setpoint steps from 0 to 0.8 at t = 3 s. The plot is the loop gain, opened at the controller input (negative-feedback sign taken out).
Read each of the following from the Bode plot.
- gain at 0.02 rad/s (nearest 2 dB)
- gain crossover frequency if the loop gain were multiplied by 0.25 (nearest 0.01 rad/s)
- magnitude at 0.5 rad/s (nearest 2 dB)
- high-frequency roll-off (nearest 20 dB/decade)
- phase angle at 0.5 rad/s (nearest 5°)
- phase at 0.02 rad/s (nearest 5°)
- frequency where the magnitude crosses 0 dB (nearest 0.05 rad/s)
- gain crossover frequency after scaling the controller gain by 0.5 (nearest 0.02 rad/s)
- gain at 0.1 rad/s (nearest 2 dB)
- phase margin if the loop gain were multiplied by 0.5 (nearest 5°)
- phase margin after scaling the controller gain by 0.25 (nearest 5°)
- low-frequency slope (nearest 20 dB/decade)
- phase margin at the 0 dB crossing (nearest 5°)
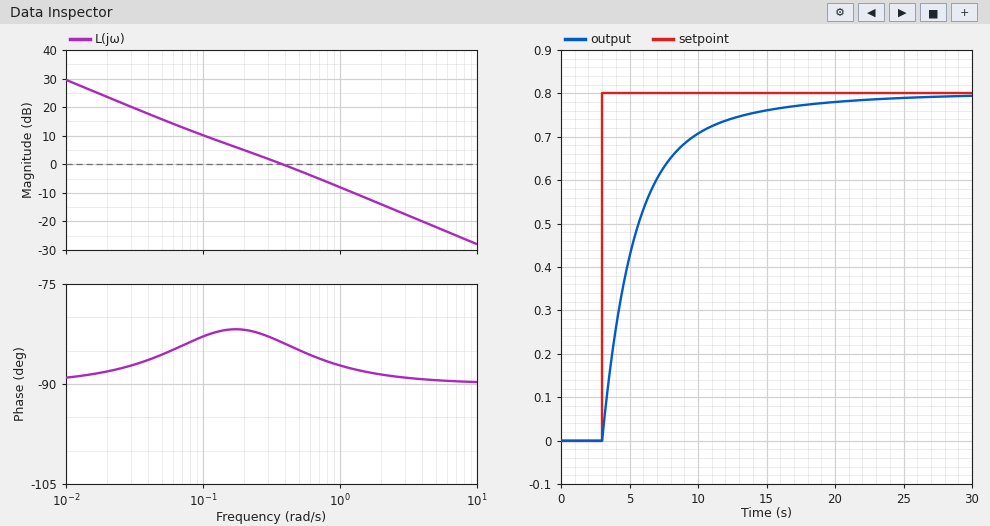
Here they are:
24 dB
0.08 rad/s
-2 dB
-20 dB/decade
-85°
-90°
0.40 rad/s
0.18 rad/s
10 dB
100°
95°
-20 dB/decade
95°
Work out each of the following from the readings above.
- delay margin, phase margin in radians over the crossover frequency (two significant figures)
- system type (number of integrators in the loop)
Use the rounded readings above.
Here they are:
4.1 s
1
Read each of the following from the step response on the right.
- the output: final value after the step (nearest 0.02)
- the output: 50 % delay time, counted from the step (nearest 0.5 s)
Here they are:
0.80
2.0 s
